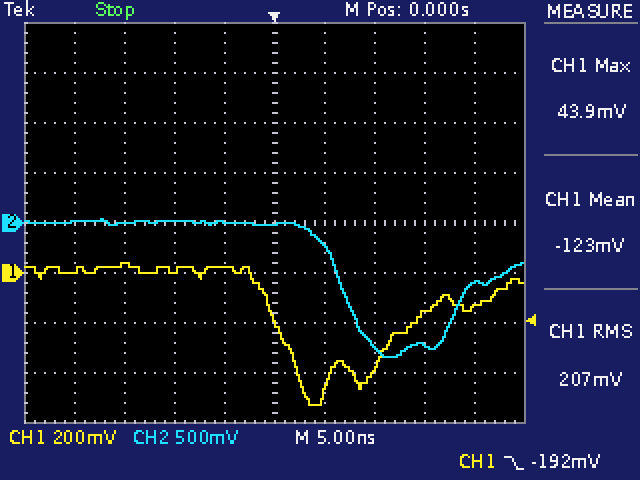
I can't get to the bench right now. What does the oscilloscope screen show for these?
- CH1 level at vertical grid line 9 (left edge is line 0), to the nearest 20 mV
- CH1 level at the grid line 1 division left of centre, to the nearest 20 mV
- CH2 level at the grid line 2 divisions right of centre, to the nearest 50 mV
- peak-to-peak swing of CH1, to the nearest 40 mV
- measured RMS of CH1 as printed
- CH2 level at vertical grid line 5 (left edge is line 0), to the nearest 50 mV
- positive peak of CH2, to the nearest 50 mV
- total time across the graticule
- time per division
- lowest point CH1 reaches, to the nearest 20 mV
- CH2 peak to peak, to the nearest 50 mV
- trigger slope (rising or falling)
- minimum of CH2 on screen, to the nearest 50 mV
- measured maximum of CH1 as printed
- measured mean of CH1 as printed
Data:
-140 mV
20 mV
-1.25 V
560 mV
207 mV
0 mV
50 mV
50 ns
5 ns
-520 mV
1.40 V
falling
-1.35 V
43.9 mV
-123 mV
